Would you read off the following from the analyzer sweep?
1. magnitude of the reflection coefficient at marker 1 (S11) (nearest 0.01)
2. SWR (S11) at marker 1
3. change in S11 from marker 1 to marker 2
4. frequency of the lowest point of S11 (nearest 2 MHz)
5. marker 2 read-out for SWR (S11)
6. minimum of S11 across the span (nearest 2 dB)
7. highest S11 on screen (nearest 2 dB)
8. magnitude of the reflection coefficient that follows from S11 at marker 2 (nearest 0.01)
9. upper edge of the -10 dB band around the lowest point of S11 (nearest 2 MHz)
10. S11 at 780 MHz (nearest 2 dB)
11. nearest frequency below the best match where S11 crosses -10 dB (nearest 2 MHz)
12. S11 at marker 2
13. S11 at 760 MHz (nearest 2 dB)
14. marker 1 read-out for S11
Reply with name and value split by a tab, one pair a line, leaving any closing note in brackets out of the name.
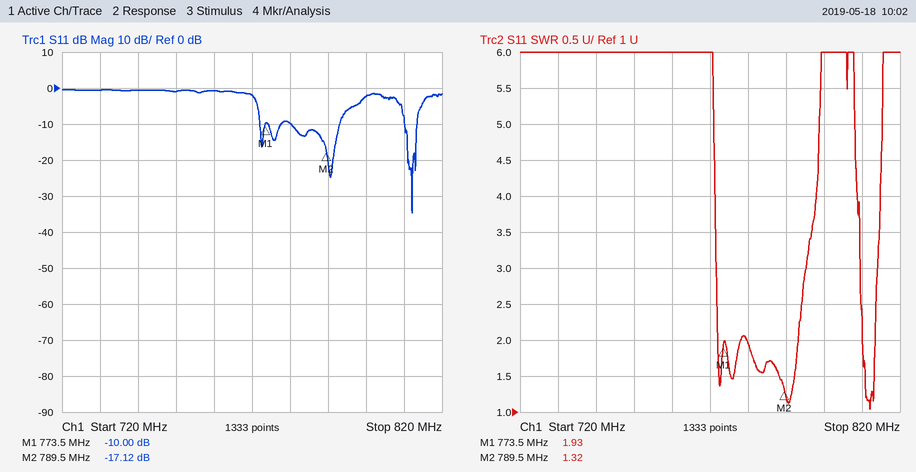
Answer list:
magnitude of the reflection coefficient at marker 1 (S11)	0.32
SWR (S11) at marker 1	1.93
change in S11 from marker 1 to marker 2	-7.12 dB
frequency of the lowest point of S11	812 MHz
marker 2 read-out for SWR	1.32
minimum of S11 across the span	-34 dB
highest S11 on screen	0 dB
magnitude of the reflection coefficient that follows from S11 at marker 2	0.14
upper edge of the -10 dB band around the lowest point of S11	814 MHz
S11 at 780 MHz	-10 dB
nearest frequency below the best match where S11 crosses -10 dB	810 MHz
S11 at marker 2	-17.12 dB
S11 at 760 MHz	0 dB
marker 1 read-out for S11	-10.00 dB
